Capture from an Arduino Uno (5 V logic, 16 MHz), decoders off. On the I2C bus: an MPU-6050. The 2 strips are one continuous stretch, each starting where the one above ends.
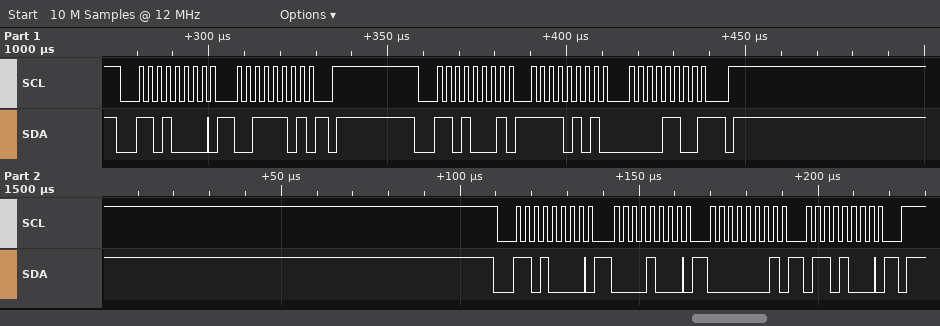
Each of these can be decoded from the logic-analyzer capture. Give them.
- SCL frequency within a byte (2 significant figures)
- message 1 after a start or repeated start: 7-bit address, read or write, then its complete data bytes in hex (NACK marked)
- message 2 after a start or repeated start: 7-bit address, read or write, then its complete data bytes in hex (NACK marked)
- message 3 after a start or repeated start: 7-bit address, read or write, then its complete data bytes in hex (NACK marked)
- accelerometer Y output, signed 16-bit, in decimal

400 kHz
0x68 write: 3D
0x68 read: F5 0C NACK
0x68 write: 08 01 68
-2804
